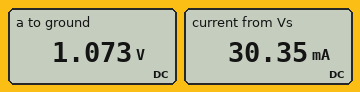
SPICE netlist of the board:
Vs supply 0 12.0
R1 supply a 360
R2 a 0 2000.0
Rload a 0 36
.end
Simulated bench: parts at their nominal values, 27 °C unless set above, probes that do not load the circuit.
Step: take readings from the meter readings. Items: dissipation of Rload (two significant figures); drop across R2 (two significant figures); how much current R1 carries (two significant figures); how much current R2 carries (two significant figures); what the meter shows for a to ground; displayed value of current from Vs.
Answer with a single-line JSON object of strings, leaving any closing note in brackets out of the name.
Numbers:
{"dissipation of Rload": "32 mW", "drop across R2": "1.1 V", "how much current R1 carries": "30 mA", "how much current R2 carries": "540 µA", "what the meter shows for a to ground": "1.073 V", "displayed value of current from Vs": "30.35 mA"}
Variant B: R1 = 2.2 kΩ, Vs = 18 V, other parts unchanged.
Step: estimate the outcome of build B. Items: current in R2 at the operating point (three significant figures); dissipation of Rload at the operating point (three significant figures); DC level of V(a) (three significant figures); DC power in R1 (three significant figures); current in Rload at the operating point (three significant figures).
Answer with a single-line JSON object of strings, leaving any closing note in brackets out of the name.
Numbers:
{"current in R2 at the operating point": "142 µA", "dissipation of Rload at the operating point": "2.25 mW", "DC level of V(a)": "285 mV", "DC power in R1": "143 mW", "current in Rload at the operating point": "7.91 mA"}
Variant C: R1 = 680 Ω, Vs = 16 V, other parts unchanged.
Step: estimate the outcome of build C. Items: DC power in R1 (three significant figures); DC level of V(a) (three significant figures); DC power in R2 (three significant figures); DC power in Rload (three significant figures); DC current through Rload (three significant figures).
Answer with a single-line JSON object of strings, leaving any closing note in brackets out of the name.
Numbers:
{"DC power in R1": "340 mW", "DC level of V(a)": "791 mV", "DC power in R2": "313 µW", "DC power in Rload": "17.4 mW", "DC current through Rload": "22.0 mA"}
